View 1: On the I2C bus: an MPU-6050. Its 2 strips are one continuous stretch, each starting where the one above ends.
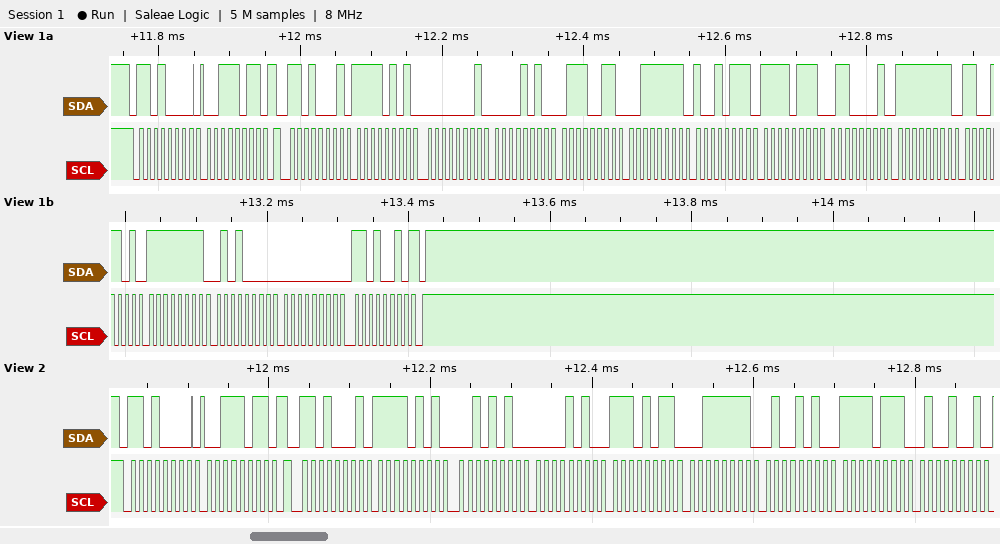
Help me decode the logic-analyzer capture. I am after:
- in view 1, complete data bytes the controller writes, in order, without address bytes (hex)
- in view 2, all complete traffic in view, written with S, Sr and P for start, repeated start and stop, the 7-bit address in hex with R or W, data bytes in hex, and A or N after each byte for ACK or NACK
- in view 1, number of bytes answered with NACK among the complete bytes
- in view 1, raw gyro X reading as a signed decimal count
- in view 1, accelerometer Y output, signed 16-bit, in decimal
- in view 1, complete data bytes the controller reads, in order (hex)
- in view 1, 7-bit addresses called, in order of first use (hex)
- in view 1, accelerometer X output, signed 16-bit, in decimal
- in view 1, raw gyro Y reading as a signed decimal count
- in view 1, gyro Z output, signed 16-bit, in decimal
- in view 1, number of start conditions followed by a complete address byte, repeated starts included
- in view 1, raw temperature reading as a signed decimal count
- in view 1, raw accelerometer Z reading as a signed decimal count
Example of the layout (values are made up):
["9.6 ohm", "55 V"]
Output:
["3B", "S 68W A 3B A Sr 68R A F5 A 2A A 0A A EB A 3F A 4A A F7 A 49 A", "1", "-51", "2675", "F5 01 0A 73 3F 97 F7 61 FF CD FF 50 00 D2", "0x68", "-2815", "-176", "210", "2", "-2207", "16279"]
